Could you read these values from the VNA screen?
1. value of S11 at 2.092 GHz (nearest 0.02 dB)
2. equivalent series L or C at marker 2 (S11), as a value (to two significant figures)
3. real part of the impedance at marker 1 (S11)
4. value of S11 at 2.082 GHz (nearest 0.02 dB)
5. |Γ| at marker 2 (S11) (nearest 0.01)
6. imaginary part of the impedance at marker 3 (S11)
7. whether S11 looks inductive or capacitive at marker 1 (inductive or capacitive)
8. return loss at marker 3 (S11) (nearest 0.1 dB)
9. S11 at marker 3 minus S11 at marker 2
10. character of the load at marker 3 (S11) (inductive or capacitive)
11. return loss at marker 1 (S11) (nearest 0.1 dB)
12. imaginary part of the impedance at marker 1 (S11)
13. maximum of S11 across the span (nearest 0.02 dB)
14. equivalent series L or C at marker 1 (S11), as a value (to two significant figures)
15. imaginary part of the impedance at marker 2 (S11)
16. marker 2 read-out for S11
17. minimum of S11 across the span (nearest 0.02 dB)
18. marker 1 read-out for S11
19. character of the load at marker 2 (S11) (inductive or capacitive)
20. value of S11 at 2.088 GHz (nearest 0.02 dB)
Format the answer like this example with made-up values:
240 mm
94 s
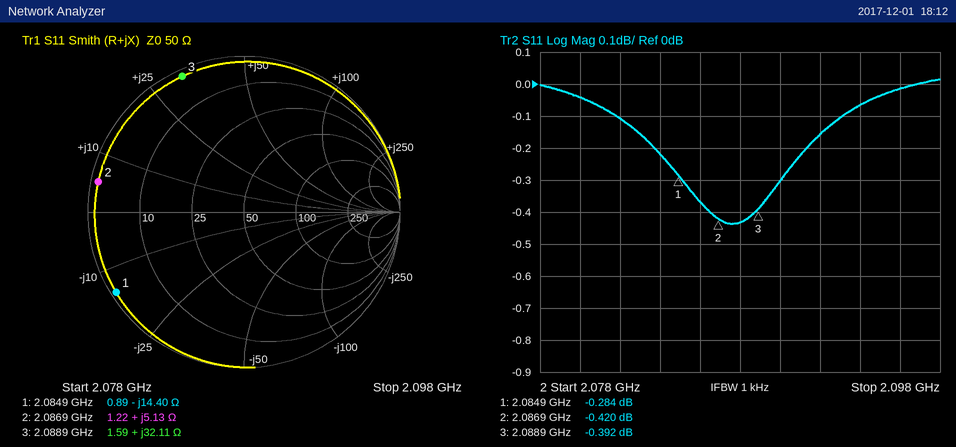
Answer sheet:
-0.16 dB
390 pH
0.89 Ω
-0.10 dB
0.95
+32.11 Ω
capacitive
0.4 dB
0.028 dB
inductive
0.3 dB
-14.40 Ω
0.02 dB
5.3 pF
+5.13 Ω
-0.420 dB
-0.44 dB
-0.284 dB
inductive
-0.44 dB
